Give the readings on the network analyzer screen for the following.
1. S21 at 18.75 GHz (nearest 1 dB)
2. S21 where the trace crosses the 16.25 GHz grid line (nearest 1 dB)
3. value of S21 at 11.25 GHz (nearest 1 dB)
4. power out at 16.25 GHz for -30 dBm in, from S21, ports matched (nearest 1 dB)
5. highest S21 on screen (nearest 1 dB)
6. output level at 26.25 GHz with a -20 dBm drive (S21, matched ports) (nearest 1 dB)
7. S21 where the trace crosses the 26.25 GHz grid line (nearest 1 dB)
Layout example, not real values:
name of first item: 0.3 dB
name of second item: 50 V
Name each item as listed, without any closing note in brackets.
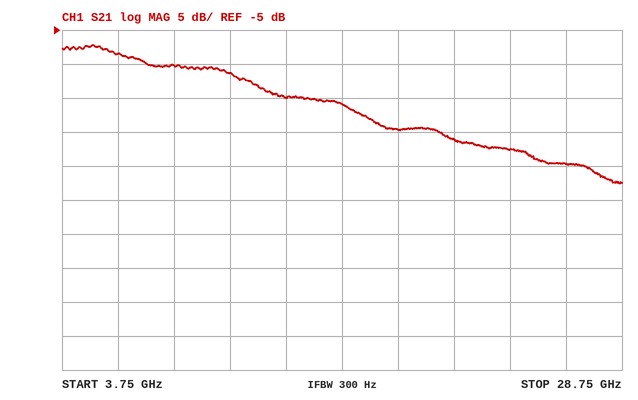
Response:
S21 at 18.75 GHz: -20 dB
S21 where the trace crosses the 16.25 GHz grid line: -16 dB
value of S21 at 11.25 GHz: -11 dB
power out at 16.25 GHz for -30 dBm in, from S21, ports matched: -46 dBm
highest S21 on screen: -7 dB
output level at 26.25 GHz with a -20 dBm drive (S21, matched ports): -45 dBm
S21 where the trace crosses the 26.25 GHz grid line: -25 dB
